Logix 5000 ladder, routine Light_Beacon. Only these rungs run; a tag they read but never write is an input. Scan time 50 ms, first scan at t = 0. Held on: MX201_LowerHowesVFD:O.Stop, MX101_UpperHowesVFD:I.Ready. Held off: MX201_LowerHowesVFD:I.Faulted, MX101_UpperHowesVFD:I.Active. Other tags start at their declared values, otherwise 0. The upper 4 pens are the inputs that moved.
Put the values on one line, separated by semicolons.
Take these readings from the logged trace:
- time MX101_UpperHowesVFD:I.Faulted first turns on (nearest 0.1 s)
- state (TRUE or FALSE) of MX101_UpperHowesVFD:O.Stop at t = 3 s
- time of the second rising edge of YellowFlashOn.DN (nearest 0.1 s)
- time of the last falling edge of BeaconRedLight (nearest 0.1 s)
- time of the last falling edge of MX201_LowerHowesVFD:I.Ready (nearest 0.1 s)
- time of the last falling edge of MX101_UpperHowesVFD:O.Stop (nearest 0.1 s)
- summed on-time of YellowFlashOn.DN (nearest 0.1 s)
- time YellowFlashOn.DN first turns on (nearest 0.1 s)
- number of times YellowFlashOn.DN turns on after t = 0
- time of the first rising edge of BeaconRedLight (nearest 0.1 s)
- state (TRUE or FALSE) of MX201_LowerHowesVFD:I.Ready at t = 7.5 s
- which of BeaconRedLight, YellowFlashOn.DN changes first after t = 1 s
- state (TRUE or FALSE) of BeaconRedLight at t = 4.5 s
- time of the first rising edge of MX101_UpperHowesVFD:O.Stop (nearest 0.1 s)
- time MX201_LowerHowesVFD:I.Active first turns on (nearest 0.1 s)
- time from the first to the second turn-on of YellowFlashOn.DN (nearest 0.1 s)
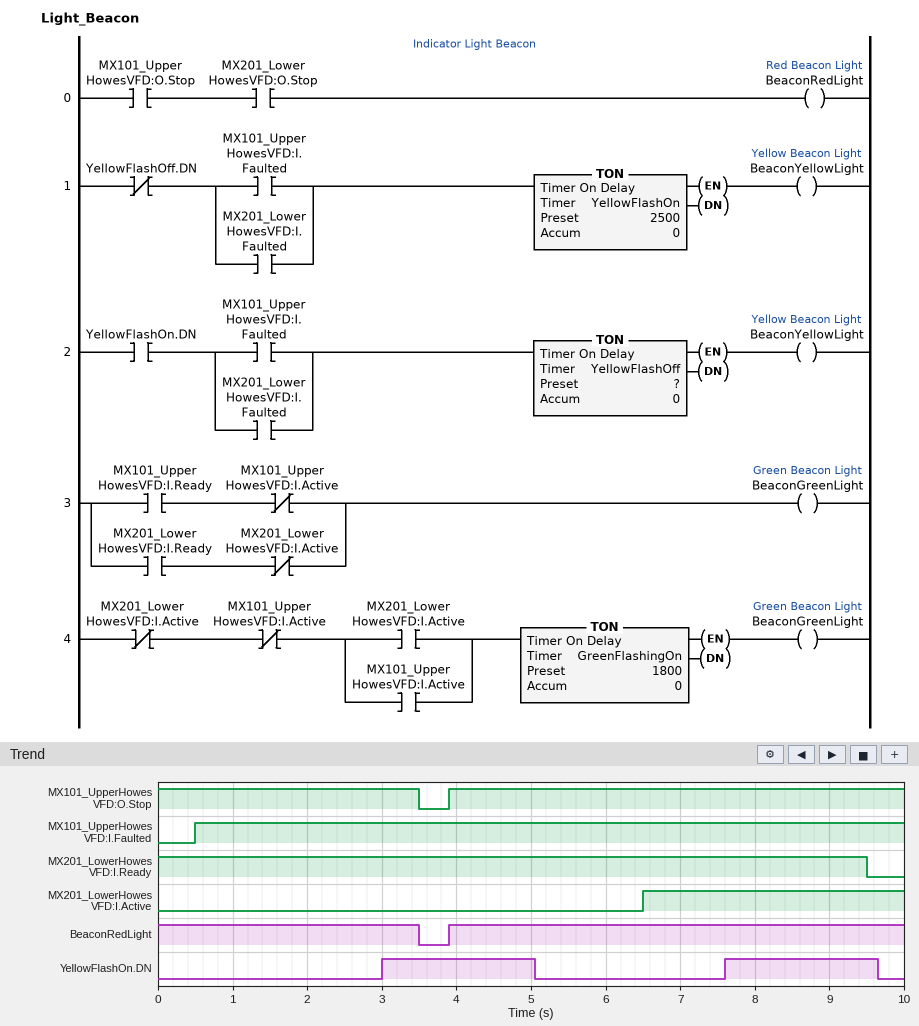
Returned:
0.5 s; TRUE; 7.6 s; 3.5 s; 9.5 s; 3.5 s; 4.1 s; 3.0 s; 2; 3.9 s; TRUE; YellowFlashOn.DN; TRUE; 3.9 s; 6.5 s; 4.6 s
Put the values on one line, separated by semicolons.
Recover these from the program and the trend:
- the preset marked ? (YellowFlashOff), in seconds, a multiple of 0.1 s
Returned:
2.0 s
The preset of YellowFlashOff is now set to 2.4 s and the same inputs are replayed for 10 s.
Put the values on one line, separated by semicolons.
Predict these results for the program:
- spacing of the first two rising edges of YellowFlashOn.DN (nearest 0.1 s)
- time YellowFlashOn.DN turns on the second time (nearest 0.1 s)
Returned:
5.0 s; 8.0 s
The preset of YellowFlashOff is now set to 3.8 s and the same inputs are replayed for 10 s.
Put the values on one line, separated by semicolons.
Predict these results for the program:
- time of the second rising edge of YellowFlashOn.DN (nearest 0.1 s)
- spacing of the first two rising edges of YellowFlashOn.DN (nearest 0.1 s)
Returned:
9.4 s; 6.4 s
